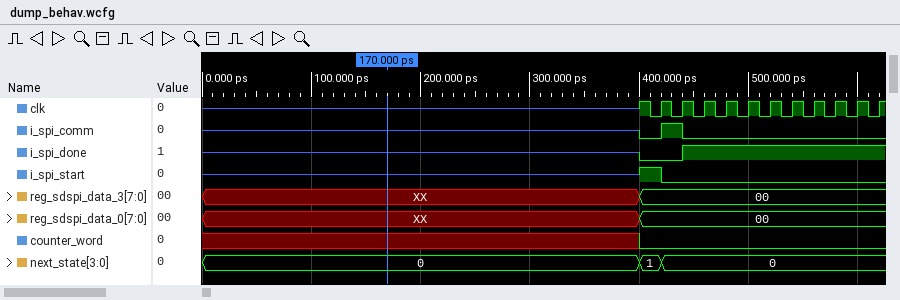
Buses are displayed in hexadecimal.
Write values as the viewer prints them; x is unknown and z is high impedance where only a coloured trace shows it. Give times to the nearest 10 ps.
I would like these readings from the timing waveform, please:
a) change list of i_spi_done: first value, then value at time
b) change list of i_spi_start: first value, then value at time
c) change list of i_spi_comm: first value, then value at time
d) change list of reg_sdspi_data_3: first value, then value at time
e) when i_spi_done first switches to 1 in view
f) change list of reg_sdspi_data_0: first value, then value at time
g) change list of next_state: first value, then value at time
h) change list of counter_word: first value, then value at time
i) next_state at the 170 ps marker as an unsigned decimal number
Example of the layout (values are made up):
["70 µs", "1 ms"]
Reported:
["z, 0 at 400 ps, 1 at 440 ps", "z, 1 at 400 ps, 0 at 420 ps", "z, 0 at 400 ps, 1 at 420 ps, 0 at 440 ps", "XX, 00 at 400 ps", "440 ps", "XX, 00 at 400 ps", "0, 1 at 400 ps, 0 at 420 ps", "x, 0 at 400 ps", "0"]
